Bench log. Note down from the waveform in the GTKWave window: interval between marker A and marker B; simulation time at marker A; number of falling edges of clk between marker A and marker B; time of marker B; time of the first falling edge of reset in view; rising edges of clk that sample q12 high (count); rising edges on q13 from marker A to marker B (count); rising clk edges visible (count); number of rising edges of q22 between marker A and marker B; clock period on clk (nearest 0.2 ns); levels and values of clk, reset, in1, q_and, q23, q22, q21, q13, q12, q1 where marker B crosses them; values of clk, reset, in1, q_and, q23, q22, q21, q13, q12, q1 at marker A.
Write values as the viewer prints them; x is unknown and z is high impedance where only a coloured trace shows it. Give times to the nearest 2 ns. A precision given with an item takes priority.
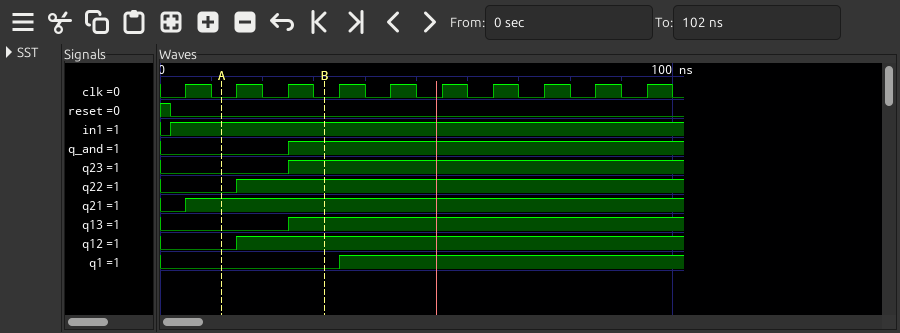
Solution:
20 ns
12 ns
2
32 ns
2 ns
8
1
10
1
10 ns
clk=0, reset=0, in1=1, q_and=1, q23=1, q22=1, q21=1, q13=1, q12=1, q1=0
clk=0, reset=0, in1=1, q_and=0, q23=0, q22=0, q21=1, q13=0, q12=0, q1=0
